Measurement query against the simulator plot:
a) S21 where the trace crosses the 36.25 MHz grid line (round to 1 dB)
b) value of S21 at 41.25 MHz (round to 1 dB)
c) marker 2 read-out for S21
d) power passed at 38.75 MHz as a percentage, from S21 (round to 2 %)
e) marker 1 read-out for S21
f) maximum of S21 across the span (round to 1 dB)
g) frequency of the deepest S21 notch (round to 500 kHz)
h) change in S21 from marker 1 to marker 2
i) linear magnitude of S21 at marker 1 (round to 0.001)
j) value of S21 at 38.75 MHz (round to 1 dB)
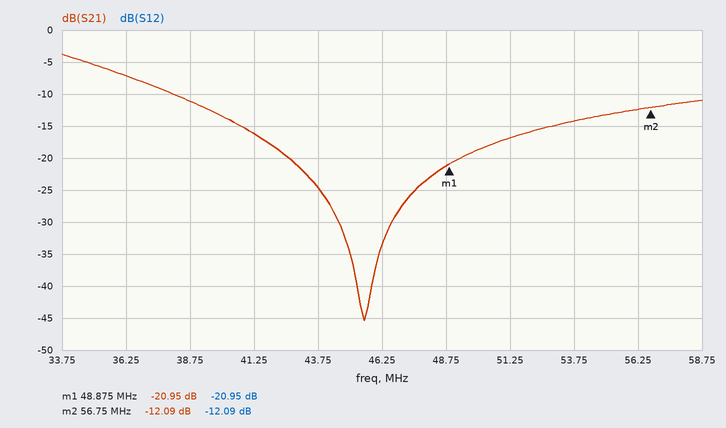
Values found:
-7 dB
-16 dB
-12.09 dB
8 %
-20.95 dB
-4 dB
45.5 MHz
8.86 dB
0.090
-11 dB
